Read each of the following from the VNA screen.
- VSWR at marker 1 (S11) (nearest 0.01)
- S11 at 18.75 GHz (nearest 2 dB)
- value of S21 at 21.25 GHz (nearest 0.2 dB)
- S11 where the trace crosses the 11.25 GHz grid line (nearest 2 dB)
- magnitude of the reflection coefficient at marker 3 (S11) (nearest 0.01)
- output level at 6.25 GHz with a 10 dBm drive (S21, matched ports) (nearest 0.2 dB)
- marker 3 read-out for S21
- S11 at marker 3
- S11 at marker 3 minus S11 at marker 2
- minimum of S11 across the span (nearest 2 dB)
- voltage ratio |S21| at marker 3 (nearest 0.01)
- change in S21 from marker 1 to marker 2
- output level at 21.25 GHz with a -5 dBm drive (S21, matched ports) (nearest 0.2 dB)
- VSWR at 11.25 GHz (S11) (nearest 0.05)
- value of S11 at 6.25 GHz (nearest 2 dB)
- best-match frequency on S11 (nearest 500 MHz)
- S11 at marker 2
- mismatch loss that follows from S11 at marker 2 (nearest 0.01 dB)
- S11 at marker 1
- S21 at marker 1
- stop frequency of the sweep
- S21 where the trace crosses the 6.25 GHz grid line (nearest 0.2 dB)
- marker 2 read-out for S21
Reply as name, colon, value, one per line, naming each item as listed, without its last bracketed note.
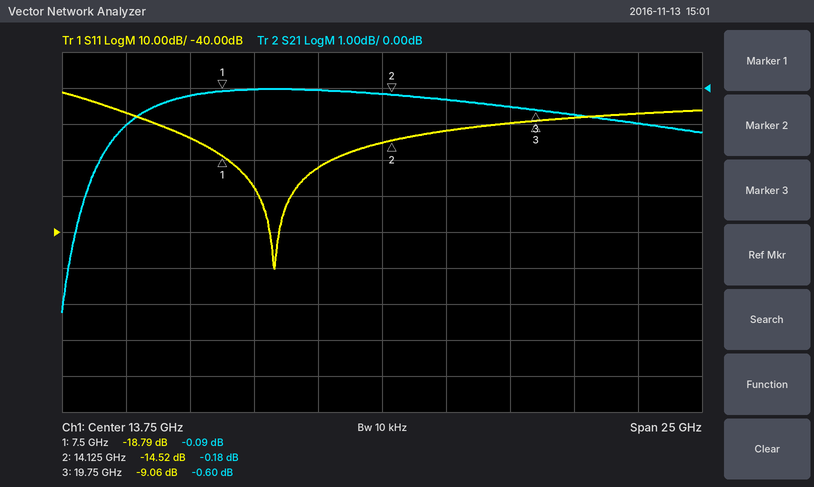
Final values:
VSWR at marker 1 (S11): 1.26
S11 at 18.75 GHz: -10 dB
value of S21 at 21.25 GHz: -0.8 dB
S11 where the trace crosses the 11.25 GHz grid line: -22 dB
magnitude of the reflection coefficient at marker 3 (S11): 0.35
output level at 6.25 GHz with a 10 dBm drive (S21, matched ports): 9.8 dBm
marker 3 read-out for S21: -0.60 dB
S11 at marker 3: -9.06 dB
S11 at marker 3 minus S11 at marker 2: 5.46 dB
minimum of S11 across the span: -50 dB
voltage ratio |S21| at marker 3: 0.93
change in S21 from marker 1 to marker 2: -0.09 dB
output level at 21.25 GHz with a -5 dBm drive (S21, matched ports): -5.8 dBm
VSWR at 11.25 GHz (S11): 1.15
value of S11 at 6.25 GHz: -14 dB
best-match frequency on S11: 9.5 GHz
S11 at marker 2: -14.52 dB
mismatch loss that follows from S11 at marker 2: 0.16 dB
S11 at marker 1: -18.79 dB
S21 at marker 1: -0.09 dB
stop frequency of the sweep: 26.25 GHz
S21 where the trace crosses the 6.25 GHz grid line: -0.2 dB
marker 2 read-out for S21: -0.18 dB
